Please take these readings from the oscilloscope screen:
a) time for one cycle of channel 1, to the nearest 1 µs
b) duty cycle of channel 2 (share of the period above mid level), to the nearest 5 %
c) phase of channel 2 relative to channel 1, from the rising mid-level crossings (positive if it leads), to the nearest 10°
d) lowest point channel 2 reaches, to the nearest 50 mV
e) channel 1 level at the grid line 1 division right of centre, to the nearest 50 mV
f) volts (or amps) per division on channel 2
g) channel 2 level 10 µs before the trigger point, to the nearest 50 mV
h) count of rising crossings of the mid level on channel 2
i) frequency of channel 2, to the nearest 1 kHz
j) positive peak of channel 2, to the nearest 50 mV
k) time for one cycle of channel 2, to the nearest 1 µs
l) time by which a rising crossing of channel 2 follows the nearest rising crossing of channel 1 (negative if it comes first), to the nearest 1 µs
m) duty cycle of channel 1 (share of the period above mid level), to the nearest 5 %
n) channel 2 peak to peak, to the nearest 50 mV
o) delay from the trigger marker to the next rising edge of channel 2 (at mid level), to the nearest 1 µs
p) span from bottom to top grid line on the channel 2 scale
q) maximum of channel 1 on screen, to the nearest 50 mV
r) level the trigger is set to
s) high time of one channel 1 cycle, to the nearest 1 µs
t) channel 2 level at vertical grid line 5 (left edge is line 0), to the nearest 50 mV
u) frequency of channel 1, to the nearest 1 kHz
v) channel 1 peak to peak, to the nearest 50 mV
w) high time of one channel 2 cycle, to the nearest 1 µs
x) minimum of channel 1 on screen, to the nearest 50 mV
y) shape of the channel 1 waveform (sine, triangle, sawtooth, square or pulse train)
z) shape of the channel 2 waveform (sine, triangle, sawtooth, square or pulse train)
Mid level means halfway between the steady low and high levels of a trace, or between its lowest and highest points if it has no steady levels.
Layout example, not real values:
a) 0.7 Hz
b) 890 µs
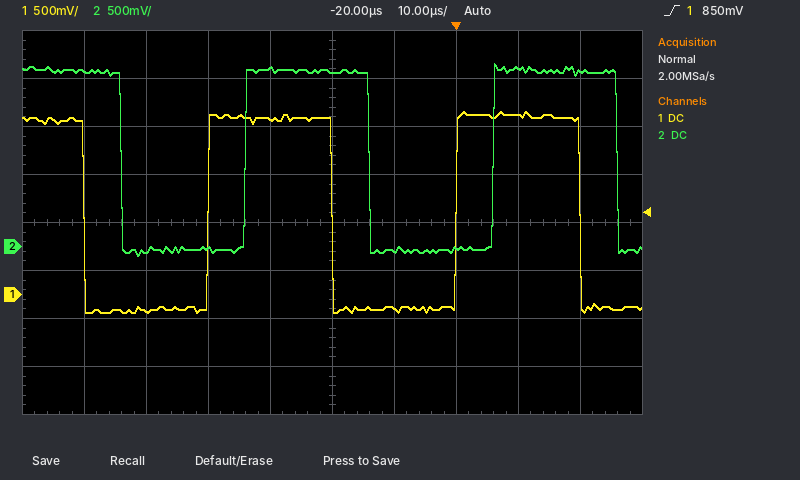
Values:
a) 40 µs
b) 50 %
c) -50°
d) -100 mV
e) -150 mV
f) 500 mV
g) -50 mV
h) 2
i) 25 kHz
j) 1.90 V
k) 40 µs
l) +6 µs
m) 50 %
n) 2.00 V
o) 6 µs
p) 4 V
q) 1.90 V
r) 850 mV
s) 20 µs
t) 1.80 V
u) 25 kHz
v) 2.10 V
w) 20 µs
x) -200 mV
y) square
z) square
